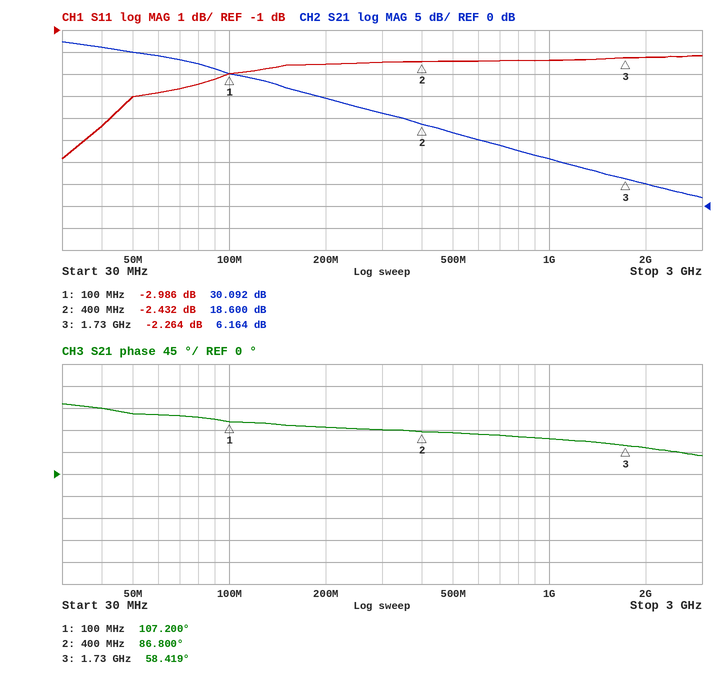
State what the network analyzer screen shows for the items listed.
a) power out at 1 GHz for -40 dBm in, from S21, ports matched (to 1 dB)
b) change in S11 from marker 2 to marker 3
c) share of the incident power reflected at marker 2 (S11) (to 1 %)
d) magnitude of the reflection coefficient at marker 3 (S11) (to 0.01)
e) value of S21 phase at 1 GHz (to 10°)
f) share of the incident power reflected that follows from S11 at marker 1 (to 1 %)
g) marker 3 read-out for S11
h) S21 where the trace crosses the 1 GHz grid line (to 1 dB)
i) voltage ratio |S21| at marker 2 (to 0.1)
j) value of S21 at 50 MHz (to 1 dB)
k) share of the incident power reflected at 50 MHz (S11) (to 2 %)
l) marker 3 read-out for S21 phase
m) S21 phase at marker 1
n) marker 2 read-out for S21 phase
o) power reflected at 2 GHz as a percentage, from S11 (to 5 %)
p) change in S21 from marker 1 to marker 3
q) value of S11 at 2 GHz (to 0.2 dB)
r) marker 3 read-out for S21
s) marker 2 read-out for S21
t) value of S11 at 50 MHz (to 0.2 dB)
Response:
-29 dBm
0.168 dB
57 %
0.77
70°
50 %
-2.264 dB
11 dB
8.5
35 dB
40 %
58.419°
107.200°
86.800°
60 %
-23.928 dB
-2.2 dB
6.164 dB
18.600 dB
-4.0 dB
